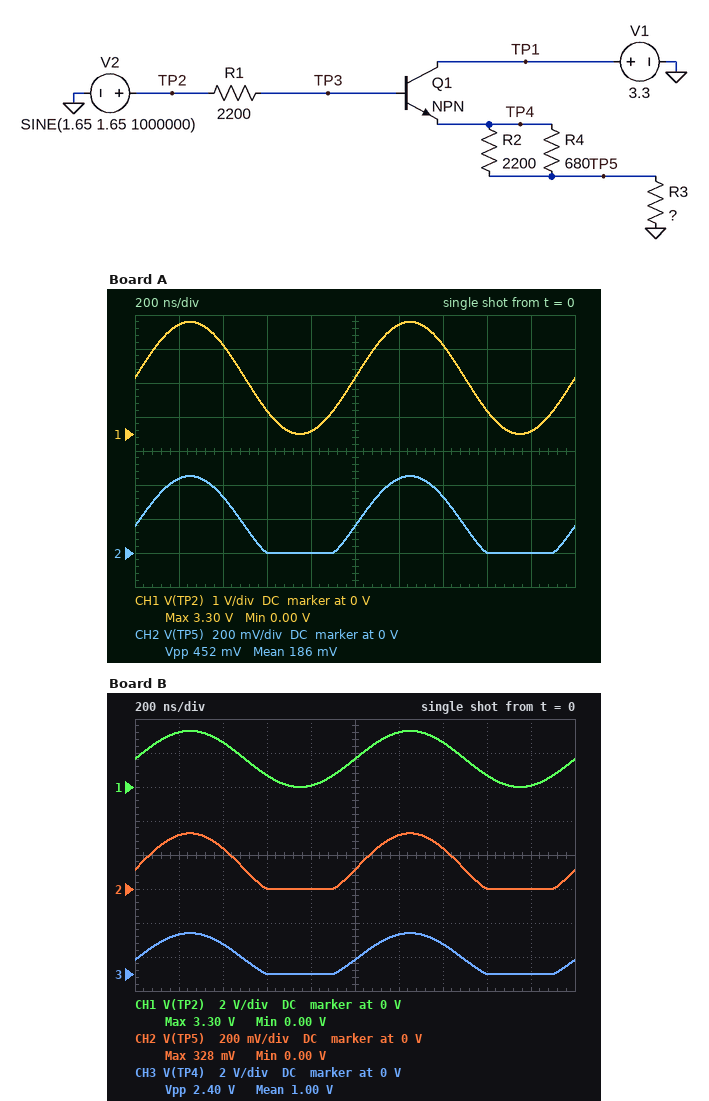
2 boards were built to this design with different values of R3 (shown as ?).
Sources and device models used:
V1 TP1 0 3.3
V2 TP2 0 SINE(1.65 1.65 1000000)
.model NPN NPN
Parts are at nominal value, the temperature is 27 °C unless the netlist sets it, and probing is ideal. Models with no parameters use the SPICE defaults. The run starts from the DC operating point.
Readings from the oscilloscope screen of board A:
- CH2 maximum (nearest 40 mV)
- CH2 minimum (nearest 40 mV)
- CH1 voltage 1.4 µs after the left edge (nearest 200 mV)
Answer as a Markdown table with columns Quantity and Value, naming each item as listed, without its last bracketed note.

| Quantity | Value |
|---|---|
| CH2 maximum | 440 mV |
| CH2 minimum | 0 V |
| CH1 voltage 1.4 µs after the left edge | 2.6 V |
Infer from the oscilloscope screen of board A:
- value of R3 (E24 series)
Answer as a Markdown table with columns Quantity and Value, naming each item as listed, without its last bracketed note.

| Quantity | Value |
|---|---|
| value of R3 | 120 Ω |
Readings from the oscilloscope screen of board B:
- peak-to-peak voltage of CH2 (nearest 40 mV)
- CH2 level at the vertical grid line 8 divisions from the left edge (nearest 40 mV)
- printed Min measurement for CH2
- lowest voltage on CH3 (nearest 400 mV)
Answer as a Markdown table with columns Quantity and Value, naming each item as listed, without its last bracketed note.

| Quantity | Value |
|---|---|
| peak-to-peak voltage of CH2 | 320 mV |
| CH2 level at the vertical grid line 8 divisions from the left edge | 0 V |
| printed Min measurement for CH2 | 0.00 V |
| lowest voltage on CH3 | 0 V |
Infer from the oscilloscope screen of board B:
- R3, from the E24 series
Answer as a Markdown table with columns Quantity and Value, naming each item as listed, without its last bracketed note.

| Quantity | Value |
|---|---|
| R3, from the E24 series | 82 Ω |
